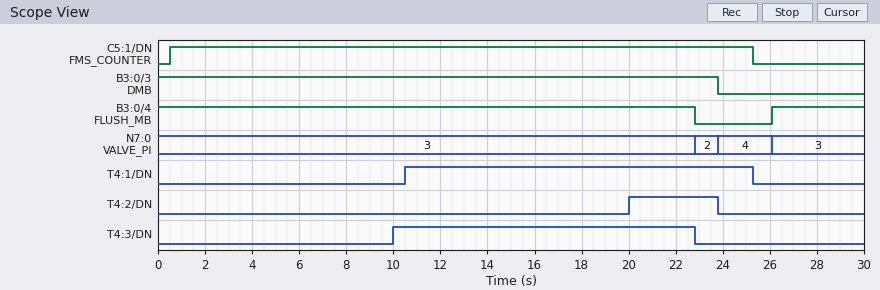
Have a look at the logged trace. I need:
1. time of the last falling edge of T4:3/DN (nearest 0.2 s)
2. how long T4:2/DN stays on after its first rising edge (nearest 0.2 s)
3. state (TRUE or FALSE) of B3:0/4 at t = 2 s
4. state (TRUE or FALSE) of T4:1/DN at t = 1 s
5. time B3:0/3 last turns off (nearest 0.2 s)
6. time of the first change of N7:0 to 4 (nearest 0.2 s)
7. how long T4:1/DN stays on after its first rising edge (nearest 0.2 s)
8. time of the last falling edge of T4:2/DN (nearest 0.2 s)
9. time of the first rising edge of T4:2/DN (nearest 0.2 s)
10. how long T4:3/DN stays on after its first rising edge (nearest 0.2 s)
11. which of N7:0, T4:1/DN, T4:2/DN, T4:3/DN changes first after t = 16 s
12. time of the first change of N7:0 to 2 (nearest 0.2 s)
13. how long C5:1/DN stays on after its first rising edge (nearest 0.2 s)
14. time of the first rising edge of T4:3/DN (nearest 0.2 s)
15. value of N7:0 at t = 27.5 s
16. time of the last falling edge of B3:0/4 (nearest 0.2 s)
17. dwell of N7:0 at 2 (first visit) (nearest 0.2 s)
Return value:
22.8 s
3.8 s
TRUE
FALSE
23.8 s
23.8 s
14.8 s
23.8 s
20.0 s
12.8 s
T4:2/DN
22.8 s
24.8 s
10.0 s
3
22.8 s
1.0 s
